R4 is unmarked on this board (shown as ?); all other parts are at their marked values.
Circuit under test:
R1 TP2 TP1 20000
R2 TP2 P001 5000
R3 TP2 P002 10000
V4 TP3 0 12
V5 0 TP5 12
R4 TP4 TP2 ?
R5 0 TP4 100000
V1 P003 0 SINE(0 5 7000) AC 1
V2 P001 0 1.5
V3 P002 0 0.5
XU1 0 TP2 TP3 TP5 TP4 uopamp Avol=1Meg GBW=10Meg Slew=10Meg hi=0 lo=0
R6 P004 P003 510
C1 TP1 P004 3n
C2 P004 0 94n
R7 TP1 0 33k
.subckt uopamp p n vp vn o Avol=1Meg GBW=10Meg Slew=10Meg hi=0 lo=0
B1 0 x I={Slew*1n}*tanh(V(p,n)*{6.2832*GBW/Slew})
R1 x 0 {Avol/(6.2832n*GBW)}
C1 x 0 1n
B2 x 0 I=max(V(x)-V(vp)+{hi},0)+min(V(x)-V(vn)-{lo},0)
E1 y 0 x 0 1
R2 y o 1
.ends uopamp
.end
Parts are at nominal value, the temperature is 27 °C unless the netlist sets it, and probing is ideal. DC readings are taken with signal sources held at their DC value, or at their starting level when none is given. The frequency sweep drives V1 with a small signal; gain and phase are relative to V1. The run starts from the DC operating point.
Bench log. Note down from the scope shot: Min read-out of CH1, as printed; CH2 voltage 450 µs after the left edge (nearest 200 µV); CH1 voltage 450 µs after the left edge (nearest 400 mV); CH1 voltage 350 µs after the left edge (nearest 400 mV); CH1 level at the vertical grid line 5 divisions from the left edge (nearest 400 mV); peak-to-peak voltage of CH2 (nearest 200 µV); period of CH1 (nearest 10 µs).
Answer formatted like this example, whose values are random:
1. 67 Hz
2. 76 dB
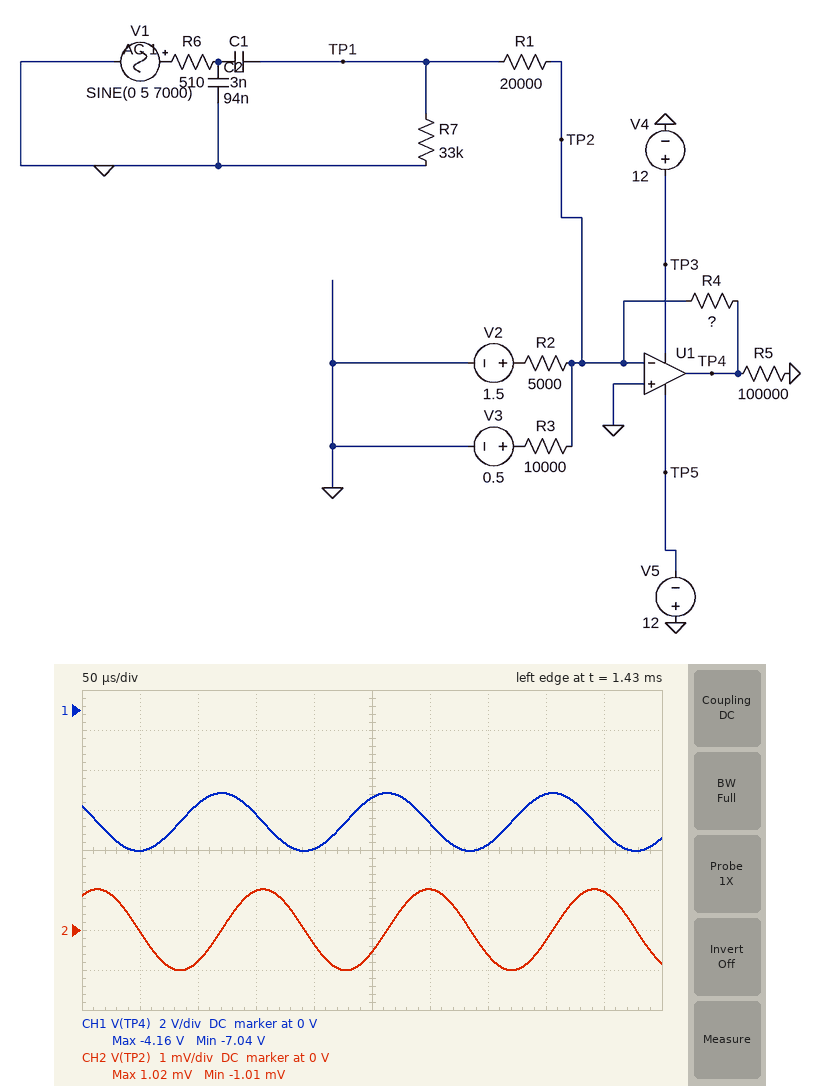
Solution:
1. -7.04 V
2. 1.0 mV
3. -6.0 V
4. -6.8 V
5. -4.4 V
6. 2.0 mV
7. 140 µs
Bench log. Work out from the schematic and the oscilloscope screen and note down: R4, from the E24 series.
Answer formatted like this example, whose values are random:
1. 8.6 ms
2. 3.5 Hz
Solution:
1. 16 kΩ
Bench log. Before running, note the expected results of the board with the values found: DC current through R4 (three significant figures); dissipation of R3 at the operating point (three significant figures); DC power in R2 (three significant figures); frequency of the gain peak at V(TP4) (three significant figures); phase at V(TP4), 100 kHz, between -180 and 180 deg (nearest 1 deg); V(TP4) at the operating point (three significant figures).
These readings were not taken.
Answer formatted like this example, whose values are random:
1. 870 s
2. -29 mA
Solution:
1. 350 µA
2. 25.0 µW
3. 450 µW
4. 3.76 kHz
5. 91 deg
6. -5.60 V
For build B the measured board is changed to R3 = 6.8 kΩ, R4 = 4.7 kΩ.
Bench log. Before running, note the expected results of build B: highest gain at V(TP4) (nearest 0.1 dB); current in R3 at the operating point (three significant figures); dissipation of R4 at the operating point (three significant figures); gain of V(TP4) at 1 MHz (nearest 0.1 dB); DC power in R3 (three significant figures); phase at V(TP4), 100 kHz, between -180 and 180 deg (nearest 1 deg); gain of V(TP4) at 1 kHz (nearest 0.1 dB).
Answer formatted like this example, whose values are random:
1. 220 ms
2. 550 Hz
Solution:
1. -19.9 dB
2. 73.5 µA
3. 656 µW
4. -62.5 dB
5. 36.8 µW
6. 93 deg
7. -25.8 dB
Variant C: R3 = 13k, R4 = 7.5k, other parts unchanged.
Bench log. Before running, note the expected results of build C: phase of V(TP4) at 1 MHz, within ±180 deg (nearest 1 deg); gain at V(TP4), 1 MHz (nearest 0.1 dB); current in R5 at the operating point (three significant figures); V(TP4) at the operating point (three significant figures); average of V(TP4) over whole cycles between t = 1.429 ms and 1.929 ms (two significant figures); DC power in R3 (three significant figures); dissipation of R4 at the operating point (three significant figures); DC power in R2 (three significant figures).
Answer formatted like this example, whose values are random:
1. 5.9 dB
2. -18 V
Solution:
1. 71 deg
2. -58.6 dB
3. 25.4 µA
4. -2.54 V
5. -2.5 V
6. 19.2 µW
7. 859 µW
8. 450 µW
